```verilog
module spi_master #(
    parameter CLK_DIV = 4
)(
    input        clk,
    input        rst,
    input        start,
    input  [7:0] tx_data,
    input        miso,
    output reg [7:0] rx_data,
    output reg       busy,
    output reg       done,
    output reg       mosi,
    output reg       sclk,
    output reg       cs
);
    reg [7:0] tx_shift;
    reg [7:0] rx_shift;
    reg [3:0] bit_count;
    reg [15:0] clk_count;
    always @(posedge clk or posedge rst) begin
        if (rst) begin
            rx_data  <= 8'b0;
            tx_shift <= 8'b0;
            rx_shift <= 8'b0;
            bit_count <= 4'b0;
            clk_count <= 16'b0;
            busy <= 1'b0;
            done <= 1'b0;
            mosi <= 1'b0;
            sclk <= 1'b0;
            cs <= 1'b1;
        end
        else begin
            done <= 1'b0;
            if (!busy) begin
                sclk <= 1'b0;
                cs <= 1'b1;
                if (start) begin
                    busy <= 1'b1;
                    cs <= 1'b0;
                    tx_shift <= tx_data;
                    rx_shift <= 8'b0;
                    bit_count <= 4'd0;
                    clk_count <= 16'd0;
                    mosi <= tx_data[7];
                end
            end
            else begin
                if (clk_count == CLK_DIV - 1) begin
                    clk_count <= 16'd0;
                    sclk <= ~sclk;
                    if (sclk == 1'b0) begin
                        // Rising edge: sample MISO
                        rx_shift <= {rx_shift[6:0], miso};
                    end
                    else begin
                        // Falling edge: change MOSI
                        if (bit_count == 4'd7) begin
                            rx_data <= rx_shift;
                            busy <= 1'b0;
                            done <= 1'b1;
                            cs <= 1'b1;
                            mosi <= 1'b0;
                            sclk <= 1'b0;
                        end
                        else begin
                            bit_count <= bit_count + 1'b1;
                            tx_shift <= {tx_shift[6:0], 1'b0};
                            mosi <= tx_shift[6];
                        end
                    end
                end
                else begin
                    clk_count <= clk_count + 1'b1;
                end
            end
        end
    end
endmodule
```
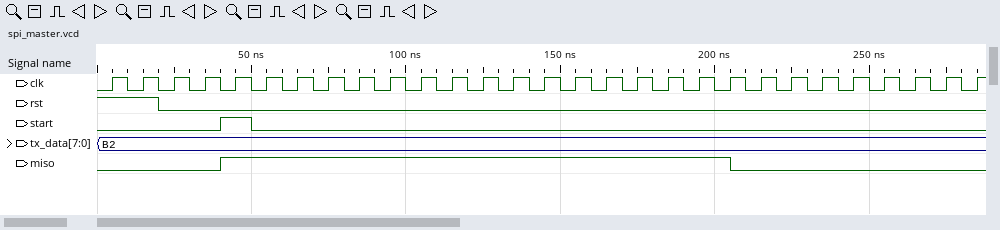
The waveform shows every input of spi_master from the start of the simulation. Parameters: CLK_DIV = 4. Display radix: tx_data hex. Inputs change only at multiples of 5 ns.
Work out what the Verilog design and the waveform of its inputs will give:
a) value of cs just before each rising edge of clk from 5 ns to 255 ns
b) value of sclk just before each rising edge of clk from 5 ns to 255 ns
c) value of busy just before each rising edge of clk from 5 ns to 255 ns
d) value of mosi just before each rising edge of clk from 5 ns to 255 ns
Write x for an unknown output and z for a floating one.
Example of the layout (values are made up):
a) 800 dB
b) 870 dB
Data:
a) 1 1 1 1 1 0 0 0 0 0 0 0 0 0 0 0 0 0 0 0 0 0 0 0 0 0
b) 0 0 0 0 0 0 0 0 0 1 1 1 1 0 0 0 0 1 1 1 1 0 0 0 0 1
c) 0 0 0 0 0 1 1 1 1 1 1 1 1 1 1 1 1 1 1 1 1 1 1 1 1 1
d) 0 0 0 0 0 1 1 1 1 1 1 1 1 0 0 0 0 0 0 0 0 1 1 1 1 1
